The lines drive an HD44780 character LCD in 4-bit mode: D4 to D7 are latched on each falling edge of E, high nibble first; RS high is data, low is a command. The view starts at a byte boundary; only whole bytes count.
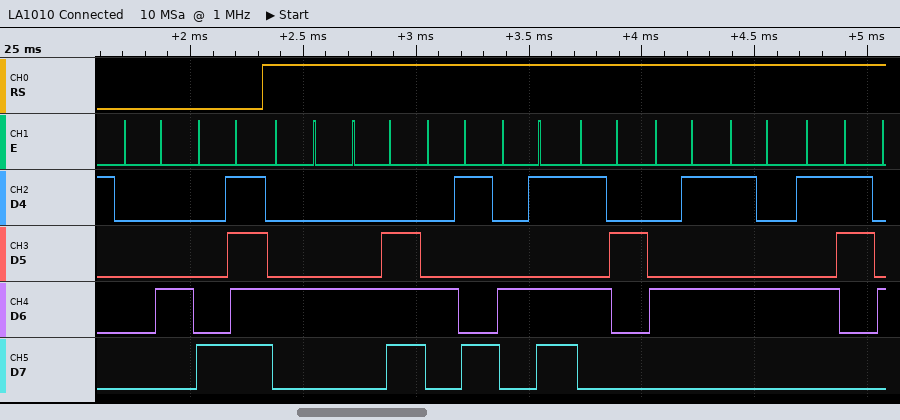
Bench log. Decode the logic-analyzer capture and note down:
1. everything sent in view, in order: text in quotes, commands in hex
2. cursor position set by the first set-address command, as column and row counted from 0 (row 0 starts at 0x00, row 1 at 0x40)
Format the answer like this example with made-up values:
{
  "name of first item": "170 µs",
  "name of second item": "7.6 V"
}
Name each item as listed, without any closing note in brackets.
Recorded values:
{
  "everything sent in view, in order: text in quotes, commands in hex": "0x04 0x8F \"DNIMRETS\"",
  "cursor position set by the first set-address command, as column and row counted from 0": "column 15, row 0"
}
